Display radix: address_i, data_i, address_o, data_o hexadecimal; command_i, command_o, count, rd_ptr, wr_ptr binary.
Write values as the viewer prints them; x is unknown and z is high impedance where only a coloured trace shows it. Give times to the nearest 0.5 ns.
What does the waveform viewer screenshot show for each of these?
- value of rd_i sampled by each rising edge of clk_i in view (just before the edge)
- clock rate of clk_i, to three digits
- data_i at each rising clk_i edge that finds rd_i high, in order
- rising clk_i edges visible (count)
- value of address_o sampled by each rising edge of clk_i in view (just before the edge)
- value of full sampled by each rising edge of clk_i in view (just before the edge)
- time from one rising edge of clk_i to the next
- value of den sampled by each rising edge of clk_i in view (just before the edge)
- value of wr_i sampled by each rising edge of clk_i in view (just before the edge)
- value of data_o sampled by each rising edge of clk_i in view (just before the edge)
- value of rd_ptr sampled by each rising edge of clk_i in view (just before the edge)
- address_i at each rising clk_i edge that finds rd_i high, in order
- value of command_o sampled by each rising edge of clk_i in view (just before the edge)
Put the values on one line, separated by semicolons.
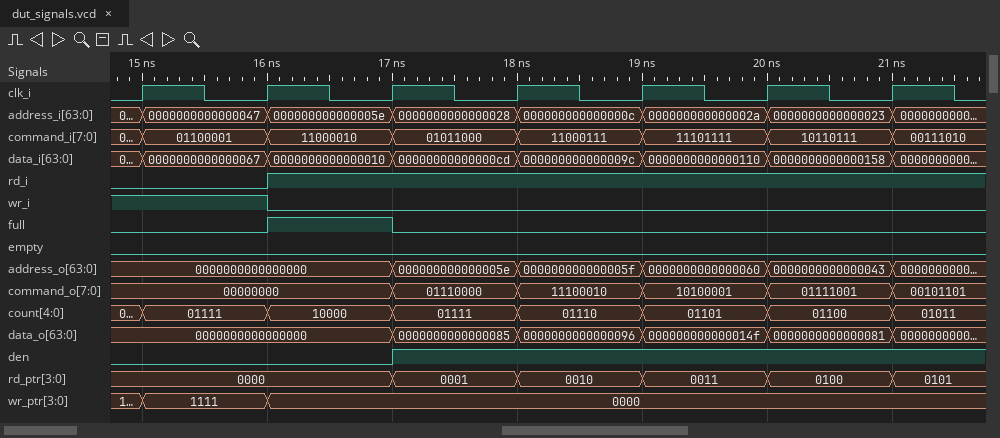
0 0 1 1 1 1 1; 1.00 GHz; 0000000000000010, 00000000000000cd, 000000000000009c, 0000000000000110, 0000000000000158; 7; 0000000000000000, 0000000000000000, 0000000000000000, 000000000000005e, 000000000000005f, 0000000000000060, 0000000000000043; 0 0 1 0 0 0 0; 1 ns; 0 0 0 1 1 1 1; 1 1 0 0 0 0 0; 0000000000000000, 0000000000000000, 0000000000000000, 0000000000000085, 0000000000000096, 000000000000014f, 0000000000000081; 0000, 0000, 0000, 0001, 0010, 0011, 0100; 000000000000005e, 0000000000000028, 000000000000000c, 000000000000002a, 0000000000000023; 00000000, 00000000, 00000000, 01110000, 11100010, 10100001, 01111001
